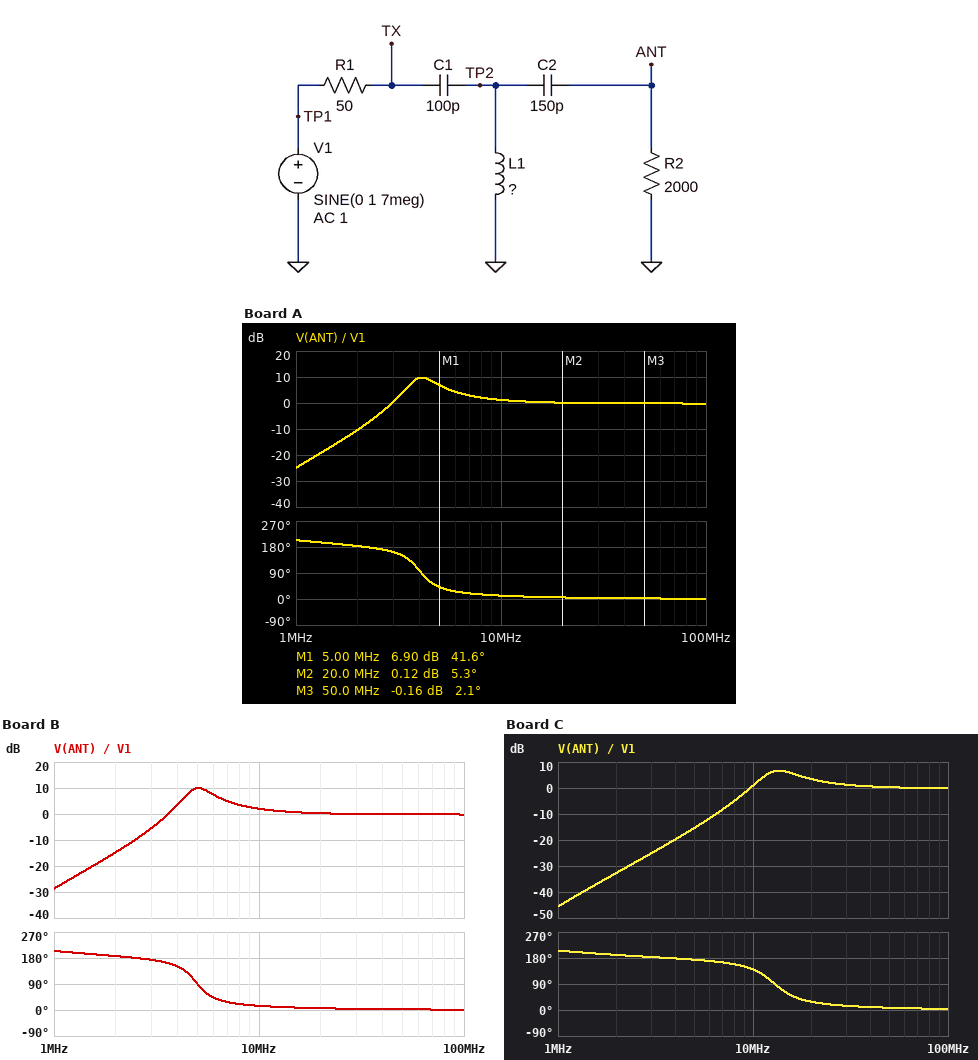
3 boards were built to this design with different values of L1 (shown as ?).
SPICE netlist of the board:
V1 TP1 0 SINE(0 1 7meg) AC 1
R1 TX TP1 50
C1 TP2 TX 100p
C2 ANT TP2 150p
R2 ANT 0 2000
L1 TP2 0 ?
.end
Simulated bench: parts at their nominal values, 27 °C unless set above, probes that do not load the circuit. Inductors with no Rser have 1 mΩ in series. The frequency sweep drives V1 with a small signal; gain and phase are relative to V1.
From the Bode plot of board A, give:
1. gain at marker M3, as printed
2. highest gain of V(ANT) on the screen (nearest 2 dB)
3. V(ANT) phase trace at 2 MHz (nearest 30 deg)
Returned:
-0.16 dB
10 dB
180 deg
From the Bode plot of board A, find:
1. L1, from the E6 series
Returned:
15 µH
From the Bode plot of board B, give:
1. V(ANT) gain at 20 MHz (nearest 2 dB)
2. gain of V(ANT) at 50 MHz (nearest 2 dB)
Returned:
0 dB
0 dB
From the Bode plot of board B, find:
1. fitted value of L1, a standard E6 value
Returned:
10 µH
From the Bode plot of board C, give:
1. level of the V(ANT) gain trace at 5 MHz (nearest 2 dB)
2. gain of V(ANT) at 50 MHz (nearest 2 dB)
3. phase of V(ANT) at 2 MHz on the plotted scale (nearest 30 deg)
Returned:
-16 dB
0 dB
180 deg
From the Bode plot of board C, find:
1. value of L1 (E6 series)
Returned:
1.5 µH
